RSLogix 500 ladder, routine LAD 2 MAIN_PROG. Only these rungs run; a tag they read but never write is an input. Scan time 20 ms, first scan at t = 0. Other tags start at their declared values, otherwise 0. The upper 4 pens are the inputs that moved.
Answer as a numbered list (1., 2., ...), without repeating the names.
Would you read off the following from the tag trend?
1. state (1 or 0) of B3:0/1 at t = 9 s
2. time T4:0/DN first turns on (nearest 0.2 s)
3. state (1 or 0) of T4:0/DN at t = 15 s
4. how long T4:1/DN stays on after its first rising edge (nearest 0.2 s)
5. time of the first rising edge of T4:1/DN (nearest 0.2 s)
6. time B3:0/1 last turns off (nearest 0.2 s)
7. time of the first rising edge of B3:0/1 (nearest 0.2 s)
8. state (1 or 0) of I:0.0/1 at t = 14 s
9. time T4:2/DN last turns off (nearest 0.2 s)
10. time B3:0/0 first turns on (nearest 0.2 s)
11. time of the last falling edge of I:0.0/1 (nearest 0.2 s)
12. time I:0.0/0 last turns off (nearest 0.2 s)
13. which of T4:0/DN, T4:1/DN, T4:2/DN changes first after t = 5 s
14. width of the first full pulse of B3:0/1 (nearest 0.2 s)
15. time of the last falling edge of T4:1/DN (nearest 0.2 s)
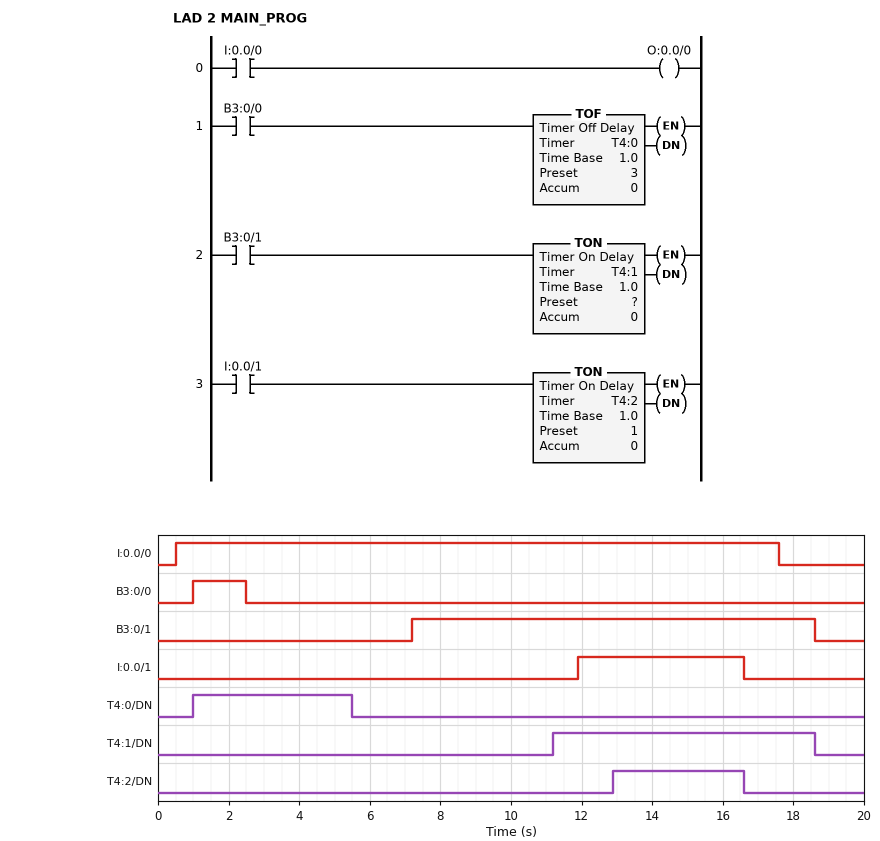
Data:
1. 1
2. 1.0 s
3. 0
4. 7.4 s
5. 11.2 s
6. 18.6 s
7. 7.2 s
8. 1
9. 16.6 s
10. 1.0 s
11. 16.6 s
12. 17.6 s
13. T4:0/DN
14. 11.4 s
15. 18.6 s
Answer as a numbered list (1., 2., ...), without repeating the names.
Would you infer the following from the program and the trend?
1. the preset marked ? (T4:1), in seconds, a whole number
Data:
1. 4 s
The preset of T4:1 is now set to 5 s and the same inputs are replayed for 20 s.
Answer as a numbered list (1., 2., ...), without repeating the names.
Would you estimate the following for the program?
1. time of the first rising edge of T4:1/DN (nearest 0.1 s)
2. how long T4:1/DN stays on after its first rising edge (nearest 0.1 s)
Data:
1. 12.2 s
2. 6.4 s
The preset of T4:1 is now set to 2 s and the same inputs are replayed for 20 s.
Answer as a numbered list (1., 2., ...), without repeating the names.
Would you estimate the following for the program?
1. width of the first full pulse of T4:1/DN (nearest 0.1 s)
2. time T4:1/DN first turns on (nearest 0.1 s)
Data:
1. 9.4 s
2. 9.2 s
